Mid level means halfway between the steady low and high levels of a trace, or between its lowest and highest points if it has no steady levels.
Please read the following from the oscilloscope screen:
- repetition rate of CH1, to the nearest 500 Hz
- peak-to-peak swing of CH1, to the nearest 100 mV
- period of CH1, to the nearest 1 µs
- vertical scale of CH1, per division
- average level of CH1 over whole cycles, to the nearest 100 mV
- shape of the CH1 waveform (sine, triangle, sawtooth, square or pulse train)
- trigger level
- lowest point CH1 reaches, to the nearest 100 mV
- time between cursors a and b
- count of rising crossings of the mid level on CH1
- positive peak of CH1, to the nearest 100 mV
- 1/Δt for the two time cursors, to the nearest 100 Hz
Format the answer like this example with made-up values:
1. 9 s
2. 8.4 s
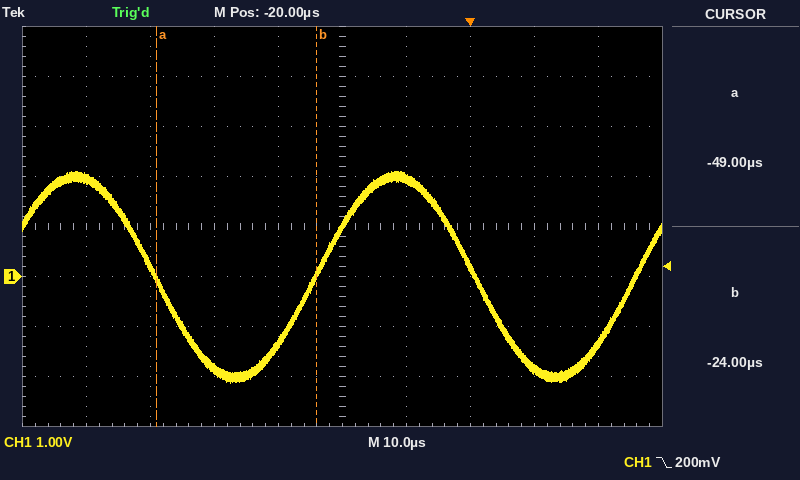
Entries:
1. 20.0 kHz
2. 4.2 V
3. 50 µs
4. 1 V
5. 0.0 V
6. sine
7. 200 mV
8. -2.1 V
9. 25 µs
10. 2
11. 2.1 V
12. 40.0 kHz
